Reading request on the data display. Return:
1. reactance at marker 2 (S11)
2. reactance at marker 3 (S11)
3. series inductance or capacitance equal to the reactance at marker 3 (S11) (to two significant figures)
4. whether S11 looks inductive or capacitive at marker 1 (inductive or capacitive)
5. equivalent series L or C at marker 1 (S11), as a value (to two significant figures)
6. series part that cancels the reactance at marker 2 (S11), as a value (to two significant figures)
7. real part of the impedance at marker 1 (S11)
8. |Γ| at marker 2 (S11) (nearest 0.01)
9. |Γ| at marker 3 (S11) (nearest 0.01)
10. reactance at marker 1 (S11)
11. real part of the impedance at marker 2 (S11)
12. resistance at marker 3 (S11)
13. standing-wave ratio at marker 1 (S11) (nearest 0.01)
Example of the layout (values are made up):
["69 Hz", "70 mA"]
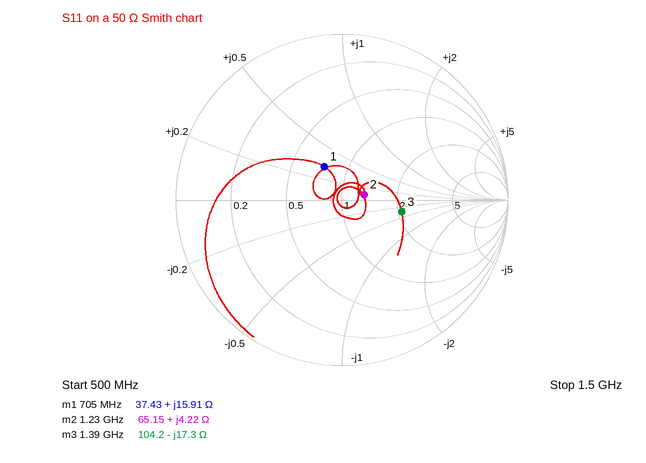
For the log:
["+4.22 Ω", "-17.3 Ω", "6.6 pF", "inductive", "3.6 nH", "31 pF", "37.43 Ω", "0.14", "0.37", "+15.91 Ω", "65.15 Ω", "104.2 Ω", "1.59"]
